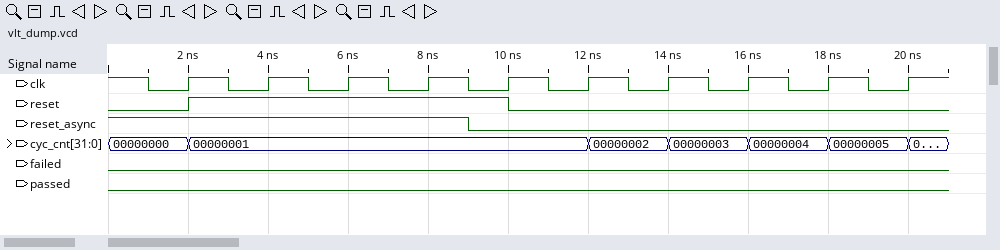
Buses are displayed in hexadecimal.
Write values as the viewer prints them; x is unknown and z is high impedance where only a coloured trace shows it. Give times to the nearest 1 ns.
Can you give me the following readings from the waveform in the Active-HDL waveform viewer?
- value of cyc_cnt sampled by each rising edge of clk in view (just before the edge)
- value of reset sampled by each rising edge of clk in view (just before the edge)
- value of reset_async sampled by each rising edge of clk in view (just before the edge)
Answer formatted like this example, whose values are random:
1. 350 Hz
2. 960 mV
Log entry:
1. 00000000, 00000001, 00000001, 00000001, 00000001, 00000001, 00000002, 00000003, 00000004, 00000005
2. 0 1 1 1 1 0 0 0 0 0
3. 1 1 1 1 0 0 0 0 0 0
